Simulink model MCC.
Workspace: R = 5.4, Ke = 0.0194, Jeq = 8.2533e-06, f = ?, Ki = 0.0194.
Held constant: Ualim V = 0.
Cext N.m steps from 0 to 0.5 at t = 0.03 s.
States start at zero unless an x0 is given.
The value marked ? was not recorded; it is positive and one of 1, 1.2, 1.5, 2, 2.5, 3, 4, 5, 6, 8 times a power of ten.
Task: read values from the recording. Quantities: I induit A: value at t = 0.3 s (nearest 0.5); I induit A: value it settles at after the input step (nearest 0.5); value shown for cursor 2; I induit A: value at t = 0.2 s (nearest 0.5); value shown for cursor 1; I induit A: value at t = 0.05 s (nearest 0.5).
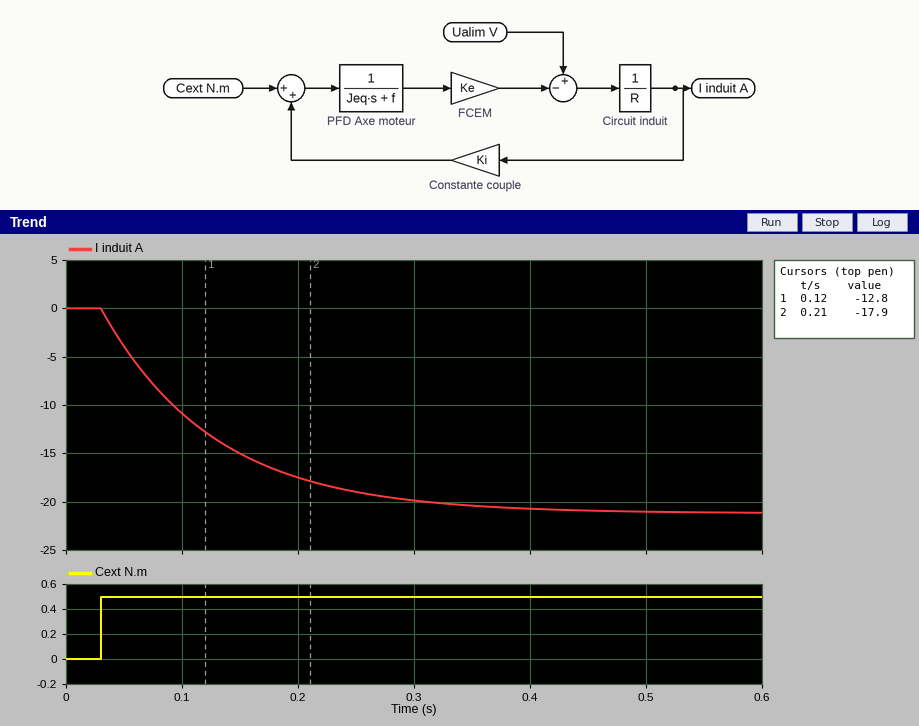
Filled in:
-20.0
-21.0
-17.9
-17.5
-12.8
-4.0
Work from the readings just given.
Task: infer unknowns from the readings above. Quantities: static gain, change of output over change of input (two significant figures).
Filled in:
-42
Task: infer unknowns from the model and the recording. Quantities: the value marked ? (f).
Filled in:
1.5e-05
